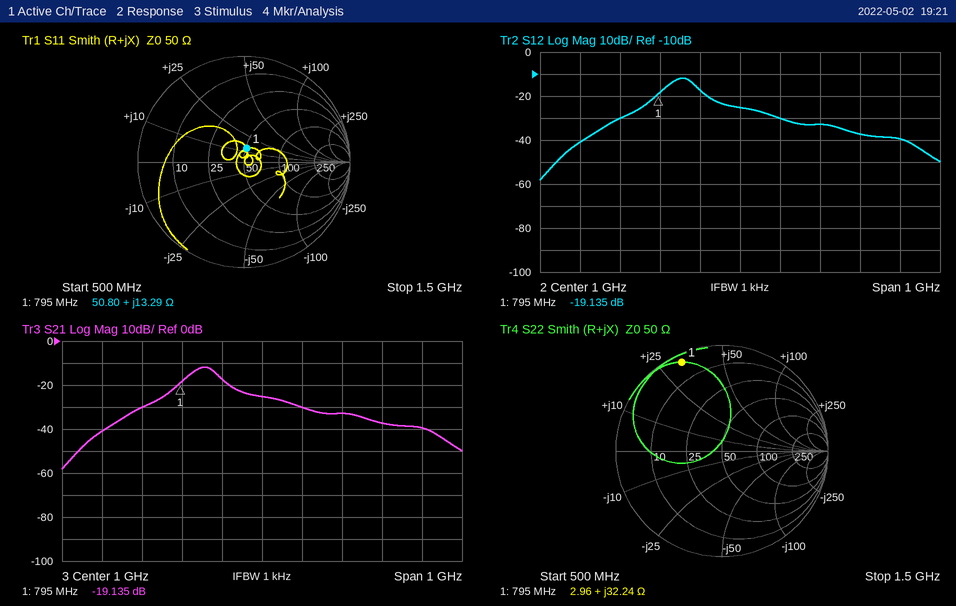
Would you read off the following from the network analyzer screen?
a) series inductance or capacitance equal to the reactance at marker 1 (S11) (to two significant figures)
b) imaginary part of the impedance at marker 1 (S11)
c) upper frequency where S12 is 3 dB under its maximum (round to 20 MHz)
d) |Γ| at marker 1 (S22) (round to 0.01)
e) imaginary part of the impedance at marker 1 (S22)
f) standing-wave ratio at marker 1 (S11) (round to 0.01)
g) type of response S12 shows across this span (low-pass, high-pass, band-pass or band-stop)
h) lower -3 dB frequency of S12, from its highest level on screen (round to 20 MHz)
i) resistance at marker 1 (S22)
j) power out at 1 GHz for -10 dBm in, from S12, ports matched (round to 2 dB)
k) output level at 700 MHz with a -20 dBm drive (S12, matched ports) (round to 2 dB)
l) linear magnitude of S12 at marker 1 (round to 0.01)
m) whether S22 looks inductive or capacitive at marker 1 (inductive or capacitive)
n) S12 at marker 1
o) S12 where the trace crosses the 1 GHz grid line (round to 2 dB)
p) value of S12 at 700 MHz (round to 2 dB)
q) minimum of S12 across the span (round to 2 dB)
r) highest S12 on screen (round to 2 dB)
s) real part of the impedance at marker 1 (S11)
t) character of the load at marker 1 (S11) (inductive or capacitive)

2.7 nH
+13.29 Ω
880 MHz
0.92
+32.24 Ω
1.30
band-pass
820 MHz
2.96 Ω
-36 dBm
-50 dBm
0.11
inductive
-19.135 dB
-26 dB
-30 dB
-58 dB
-12 dB
50.80 Ω
inductive
